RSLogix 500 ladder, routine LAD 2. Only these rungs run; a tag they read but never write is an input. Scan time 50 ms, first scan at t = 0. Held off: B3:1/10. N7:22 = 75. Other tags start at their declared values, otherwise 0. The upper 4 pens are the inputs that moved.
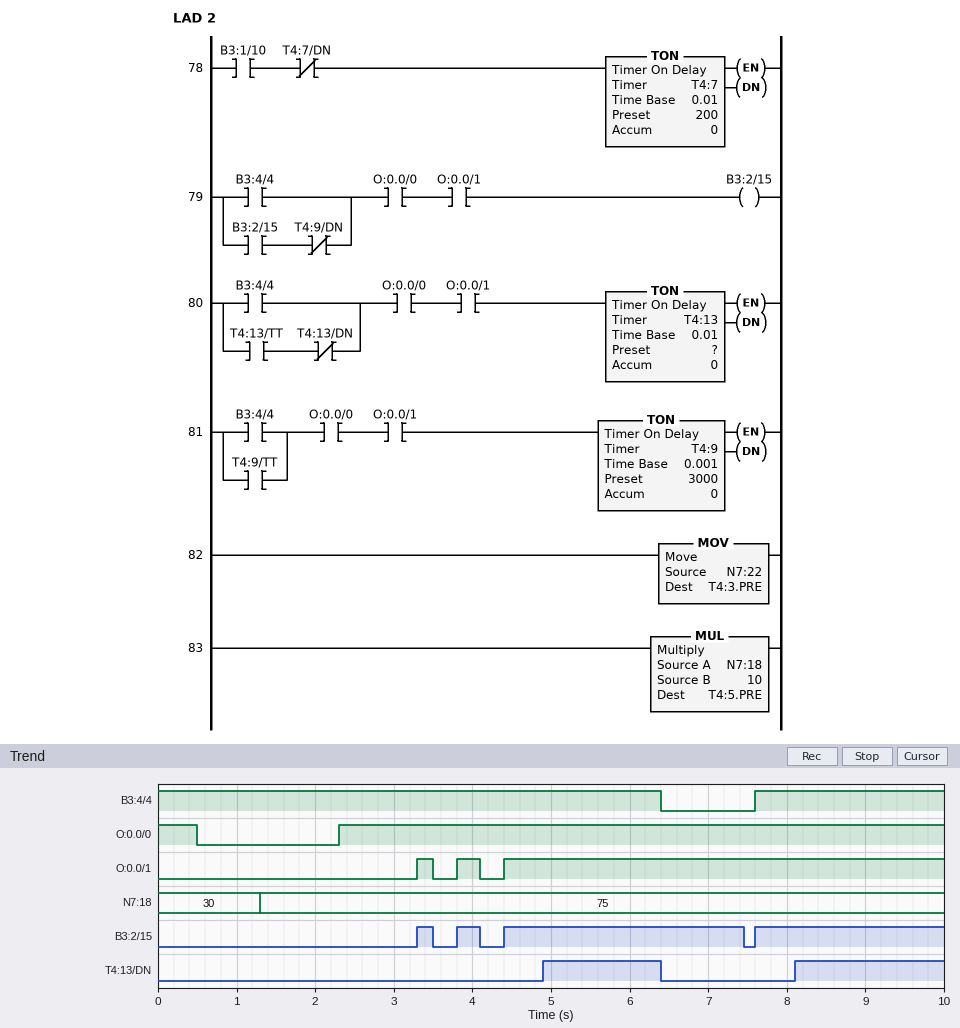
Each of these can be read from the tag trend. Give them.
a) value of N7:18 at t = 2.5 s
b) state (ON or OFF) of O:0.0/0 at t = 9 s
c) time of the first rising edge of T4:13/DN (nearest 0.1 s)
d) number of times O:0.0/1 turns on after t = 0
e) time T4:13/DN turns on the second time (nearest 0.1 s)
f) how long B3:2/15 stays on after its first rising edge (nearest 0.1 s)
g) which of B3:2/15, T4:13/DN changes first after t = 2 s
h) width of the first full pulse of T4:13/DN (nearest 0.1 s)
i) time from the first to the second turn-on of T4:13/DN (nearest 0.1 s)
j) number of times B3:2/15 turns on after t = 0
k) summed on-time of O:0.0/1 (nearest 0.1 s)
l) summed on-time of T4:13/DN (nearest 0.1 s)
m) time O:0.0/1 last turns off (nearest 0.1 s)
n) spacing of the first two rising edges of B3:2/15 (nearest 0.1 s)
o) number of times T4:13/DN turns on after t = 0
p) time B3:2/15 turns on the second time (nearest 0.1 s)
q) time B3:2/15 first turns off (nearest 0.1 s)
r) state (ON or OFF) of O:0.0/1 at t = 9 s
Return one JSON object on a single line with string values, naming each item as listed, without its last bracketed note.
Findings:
{"value of N7:18 at t = 2.5 s": "75", "state (ON or OFF) of O:0.0/0 at t = 9 s": "ON", "time of the first rising edge of T4:13/DN": "4.9 s", "number of times O:0.0/1 turns on after t = 0": "3", "time T4:13/DN turns on the second time": "8.1 s", "how long B3:2/15 stays on after its first rising edge": "0.2 s", "which of B3:2/15, T4:13/DN changes first after t = 2 s": "B3:2/15", "width of the first full pulse of T4:13/DN": "1.5 s", "time from the first to the second turn-on of T4:13/DN": "3.2 s", "number of times B3:2/15 turns on after t = 0": "4", "summed on-time of O:0.0/1": "6.1 s", "summed on-time of T4:13/DN": "3.4 s", "time O:0.0/1 last turns off": "4.1 s", "spacing of the first two rising edges of B3:2/15": "0.5 s", "number of times T4:13/DN turns on after t = 0": "2", "time B3:2/15 turns on the second time": "3.8 s", "time B3:2/15 first turns off": "3.5 s", "state (ON or OFF) of O:0.0/1 at t = 9 s": "ON"}
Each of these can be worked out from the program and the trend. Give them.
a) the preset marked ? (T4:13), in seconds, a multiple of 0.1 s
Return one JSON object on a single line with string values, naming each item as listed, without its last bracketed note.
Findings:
{"the preset marked ? (T4:13), in seconds, a multiple of 0.1 s": "0.5 s"}
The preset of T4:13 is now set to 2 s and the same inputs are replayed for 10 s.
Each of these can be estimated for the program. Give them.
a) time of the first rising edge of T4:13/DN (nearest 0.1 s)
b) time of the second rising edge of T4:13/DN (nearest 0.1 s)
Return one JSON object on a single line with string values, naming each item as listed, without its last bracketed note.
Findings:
{"time of the first rising edge of T4:13/DN": "6.4 s", "time of the second rising edge of T4:13/DN": "9.6 s"}
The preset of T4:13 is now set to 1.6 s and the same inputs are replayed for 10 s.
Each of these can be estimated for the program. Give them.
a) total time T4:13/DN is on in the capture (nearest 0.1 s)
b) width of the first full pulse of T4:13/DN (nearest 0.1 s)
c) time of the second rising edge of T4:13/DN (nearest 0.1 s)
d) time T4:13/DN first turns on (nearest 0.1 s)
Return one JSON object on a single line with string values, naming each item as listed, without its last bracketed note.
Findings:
{"total time T4:13/DN is on in the capture": "1.2 s", "width of the first full pulse of T4:13/DN": "0.4 s", "time of the second rising edge of T4:13/DN": "9.2 s", "time T4:13/DN first turns on": "6.0 s"}
